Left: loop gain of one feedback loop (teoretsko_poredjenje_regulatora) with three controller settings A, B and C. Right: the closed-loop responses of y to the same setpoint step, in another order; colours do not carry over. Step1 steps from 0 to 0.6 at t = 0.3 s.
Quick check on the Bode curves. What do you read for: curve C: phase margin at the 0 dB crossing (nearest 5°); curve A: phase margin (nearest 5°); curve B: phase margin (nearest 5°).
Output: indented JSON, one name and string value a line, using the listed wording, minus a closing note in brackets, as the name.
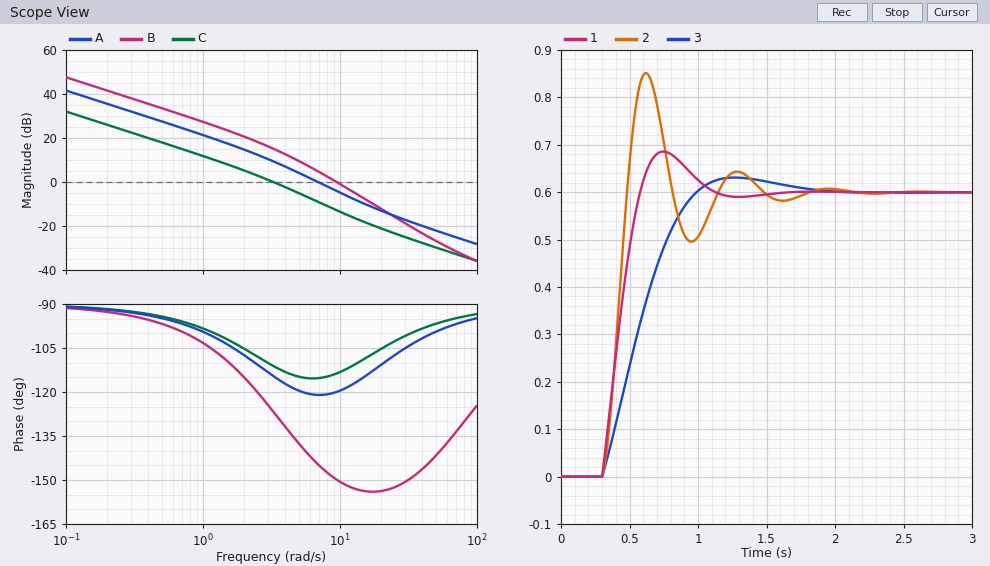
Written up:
{
  "curve C: phase margin at the 0 dB crossing": "70°",
  "curve A: phase margin": "60°",
  "curve B: phase margin": "30°"
}
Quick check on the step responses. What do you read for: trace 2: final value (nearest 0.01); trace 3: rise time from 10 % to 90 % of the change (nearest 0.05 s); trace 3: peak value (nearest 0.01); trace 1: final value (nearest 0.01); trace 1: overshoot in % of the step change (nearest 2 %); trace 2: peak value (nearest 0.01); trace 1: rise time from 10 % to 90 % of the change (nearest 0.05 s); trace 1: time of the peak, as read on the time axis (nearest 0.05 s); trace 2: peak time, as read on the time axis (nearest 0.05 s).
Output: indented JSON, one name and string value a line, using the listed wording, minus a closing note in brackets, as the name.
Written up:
{
  "trace 2: final value": "0.60",
  "trace 3: rise time from 10 % to 90 % of the change": "0.50 s",
  "trace 3: peak value": "0.63",
  "trace 1: final value": "0.60",
  "trace 1: overshoot in % of the step change": "14 %",
  "trace 2: peak value": "0.85",
  "trace 1: rise time from 10 % to 90 % of the change": "0.20 s",
  "trace 1: time of the peak, as read on the time axis": "0.75 s",
  "trace 2: peak time, as read on the time axis": "0.60 s"
}
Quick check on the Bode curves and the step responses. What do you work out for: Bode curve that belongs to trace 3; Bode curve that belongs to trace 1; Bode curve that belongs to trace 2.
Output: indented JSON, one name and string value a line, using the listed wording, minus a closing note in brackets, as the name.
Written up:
{
  "Bode curve that belongs to trace 3": "C",
  "Bode curve that belongs to trace 1": "A",
  "Bode curve that belongs to trace 2": "B"
}
